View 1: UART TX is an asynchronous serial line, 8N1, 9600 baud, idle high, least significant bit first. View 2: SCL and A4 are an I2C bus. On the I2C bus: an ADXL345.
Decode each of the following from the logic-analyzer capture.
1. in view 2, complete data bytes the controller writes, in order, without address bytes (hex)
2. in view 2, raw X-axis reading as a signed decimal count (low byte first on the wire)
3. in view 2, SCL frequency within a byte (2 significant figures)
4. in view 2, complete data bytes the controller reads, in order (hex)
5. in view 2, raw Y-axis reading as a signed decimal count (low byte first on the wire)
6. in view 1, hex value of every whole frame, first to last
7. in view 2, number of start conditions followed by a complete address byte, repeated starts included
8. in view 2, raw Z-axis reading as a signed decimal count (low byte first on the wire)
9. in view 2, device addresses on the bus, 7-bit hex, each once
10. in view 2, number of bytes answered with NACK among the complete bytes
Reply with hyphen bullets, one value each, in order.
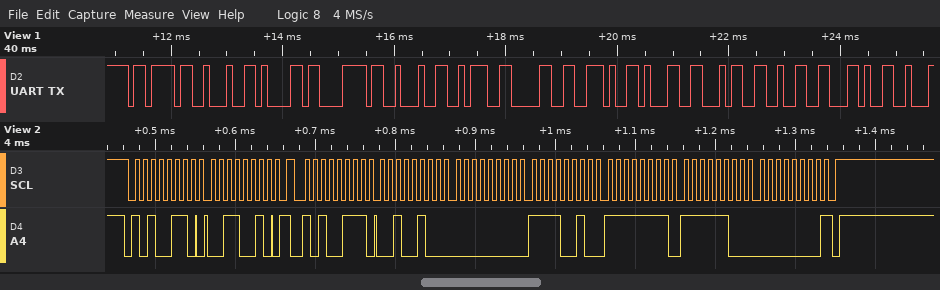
- 32
- 36
- 100 kHz
- 24 00 F2 FF FC 00
- -14
- 7B 22 61 78 22 3A 30 2E 31 34 32 2C
- 2
- 252
- 0x53
- 1
